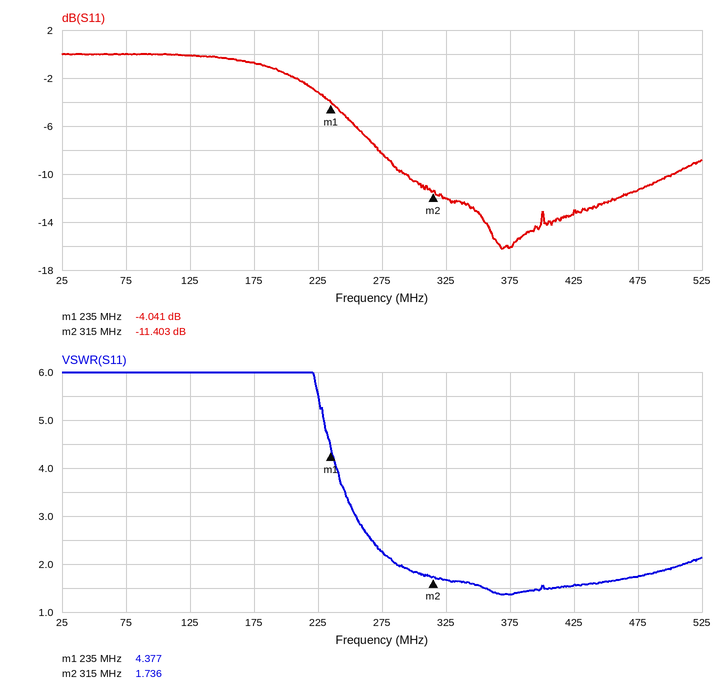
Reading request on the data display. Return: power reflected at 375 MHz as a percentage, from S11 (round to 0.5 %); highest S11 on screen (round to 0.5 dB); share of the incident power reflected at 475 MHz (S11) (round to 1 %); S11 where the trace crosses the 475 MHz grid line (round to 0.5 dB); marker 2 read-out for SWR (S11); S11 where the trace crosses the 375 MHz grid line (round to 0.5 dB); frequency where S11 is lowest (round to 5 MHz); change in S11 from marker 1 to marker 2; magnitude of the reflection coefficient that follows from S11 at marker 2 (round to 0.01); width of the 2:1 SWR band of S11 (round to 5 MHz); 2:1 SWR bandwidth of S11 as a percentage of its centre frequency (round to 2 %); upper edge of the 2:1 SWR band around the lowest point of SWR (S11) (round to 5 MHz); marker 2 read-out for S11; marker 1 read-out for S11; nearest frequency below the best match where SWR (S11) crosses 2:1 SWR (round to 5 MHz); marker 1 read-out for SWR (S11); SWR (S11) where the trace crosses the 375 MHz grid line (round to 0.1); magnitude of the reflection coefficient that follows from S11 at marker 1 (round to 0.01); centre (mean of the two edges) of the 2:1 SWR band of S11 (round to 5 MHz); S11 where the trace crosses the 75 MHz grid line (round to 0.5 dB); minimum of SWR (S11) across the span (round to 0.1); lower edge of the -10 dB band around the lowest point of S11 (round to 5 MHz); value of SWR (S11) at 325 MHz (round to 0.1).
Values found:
2.5 %
0.0 dB
7 %
-11.5 dB
1.736
-16.0 dB
370 MHz
-7.362 dB
0.27
225 MHz
56 %
510 MHz
-11.403 dB
-4.041 dB
285 MHz
4.377
1.4
0.63
400 MHz
0.0 dB
1.4
295 MHz
1.7
